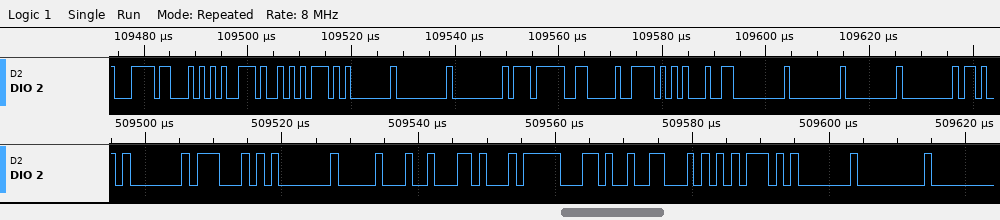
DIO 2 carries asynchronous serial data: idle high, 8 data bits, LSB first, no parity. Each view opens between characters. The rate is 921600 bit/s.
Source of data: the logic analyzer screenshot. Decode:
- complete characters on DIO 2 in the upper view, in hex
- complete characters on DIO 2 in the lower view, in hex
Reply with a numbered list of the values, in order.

1. BC, 54, 2E, 75, 01, 00, 00, F7, 06, 5E, 91, 00, 00, 00, 00
2. 01, 47, 01, 10, 62, F4, 2C, 46, 75, 01, 00
